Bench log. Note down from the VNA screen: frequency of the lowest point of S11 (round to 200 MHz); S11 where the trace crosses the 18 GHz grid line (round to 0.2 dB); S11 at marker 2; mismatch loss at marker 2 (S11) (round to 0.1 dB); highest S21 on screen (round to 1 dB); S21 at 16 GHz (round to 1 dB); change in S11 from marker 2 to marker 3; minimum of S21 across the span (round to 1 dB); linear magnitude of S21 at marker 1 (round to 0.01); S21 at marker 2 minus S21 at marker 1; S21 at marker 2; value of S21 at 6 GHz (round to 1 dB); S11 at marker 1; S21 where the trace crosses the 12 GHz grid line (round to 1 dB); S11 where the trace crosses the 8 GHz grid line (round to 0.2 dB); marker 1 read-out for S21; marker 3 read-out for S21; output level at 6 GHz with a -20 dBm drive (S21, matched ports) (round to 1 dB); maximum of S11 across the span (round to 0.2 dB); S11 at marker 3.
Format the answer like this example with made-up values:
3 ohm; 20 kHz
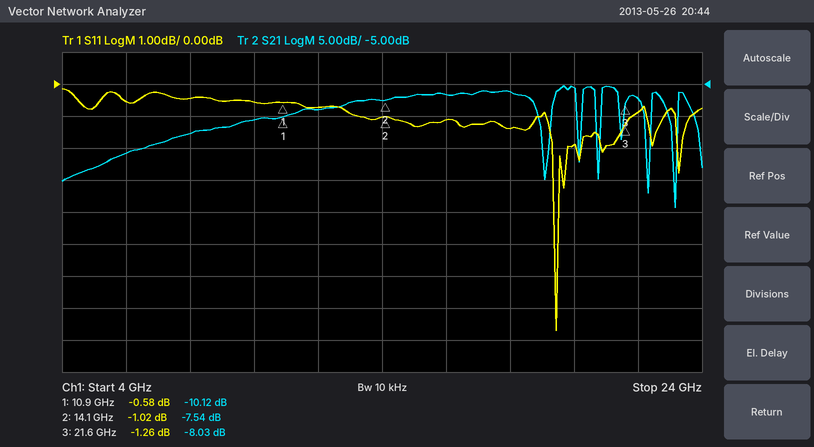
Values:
19.4 GHz; -1.4 dB; -1.02 dB; 6.8 dB; -5 dB; -7 dB; -0.24 dB; -24 dB; 0.31; 2.58 dB; -7.54 dB; -16 dB; -0.58 dB; -9 dB; -0.4 dB; -10.12 dB; -8.03 dB; -36 dBm; -0.2 dB; -1.26 dB
